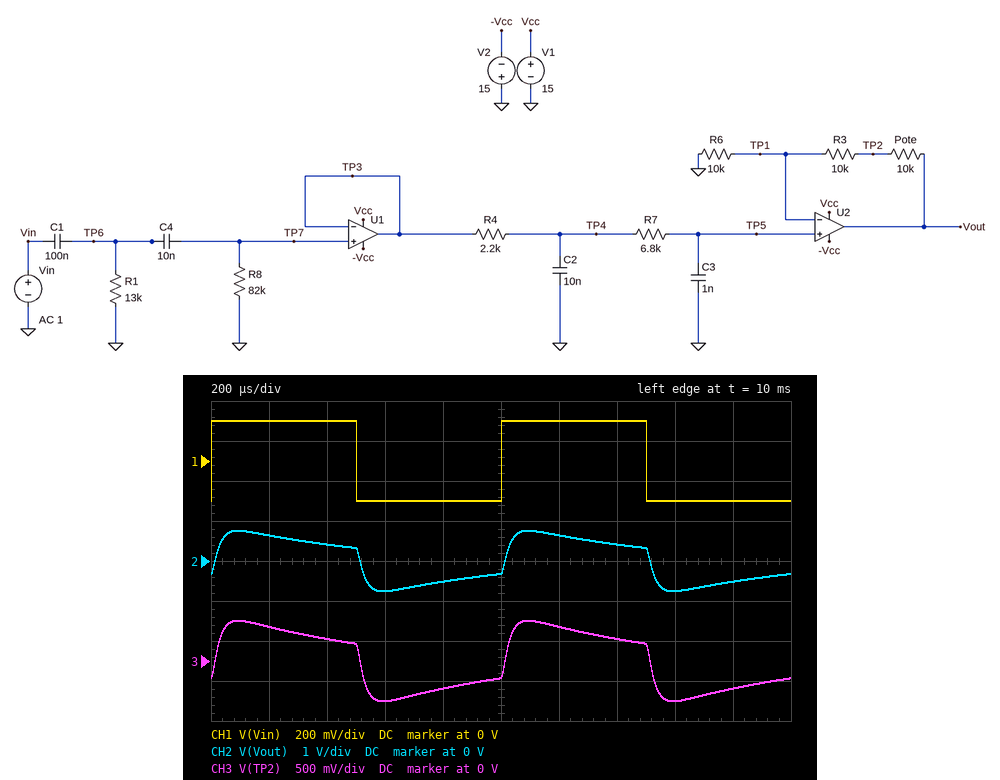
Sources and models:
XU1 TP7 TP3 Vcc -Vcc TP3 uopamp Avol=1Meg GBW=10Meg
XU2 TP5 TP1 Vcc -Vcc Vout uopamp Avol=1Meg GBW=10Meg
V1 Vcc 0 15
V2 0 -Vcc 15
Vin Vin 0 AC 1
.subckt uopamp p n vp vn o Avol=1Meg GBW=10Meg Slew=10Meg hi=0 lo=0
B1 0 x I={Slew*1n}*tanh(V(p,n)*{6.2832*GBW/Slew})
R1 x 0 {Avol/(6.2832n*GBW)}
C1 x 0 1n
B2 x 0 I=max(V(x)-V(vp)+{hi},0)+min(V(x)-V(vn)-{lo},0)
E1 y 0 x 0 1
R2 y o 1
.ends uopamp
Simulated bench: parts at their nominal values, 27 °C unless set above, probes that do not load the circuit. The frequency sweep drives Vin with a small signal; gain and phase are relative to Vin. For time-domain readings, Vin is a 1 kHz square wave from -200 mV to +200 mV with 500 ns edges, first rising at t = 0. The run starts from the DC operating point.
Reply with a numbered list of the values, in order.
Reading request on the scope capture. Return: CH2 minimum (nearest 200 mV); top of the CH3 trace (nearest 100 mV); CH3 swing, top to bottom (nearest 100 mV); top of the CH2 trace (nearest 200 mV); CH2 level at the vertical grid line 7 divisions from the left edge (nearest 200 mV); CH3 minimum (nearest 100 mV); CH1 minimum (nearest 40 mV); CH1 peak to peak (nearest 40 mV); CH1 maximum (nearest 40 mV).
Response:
1. -800 mV
2. 500 mV
3. 1.0 V
4. 800 mV
5. 400 mV
6. -500 mV
7. -200 mV
8. 400 mV
9. 200 mV
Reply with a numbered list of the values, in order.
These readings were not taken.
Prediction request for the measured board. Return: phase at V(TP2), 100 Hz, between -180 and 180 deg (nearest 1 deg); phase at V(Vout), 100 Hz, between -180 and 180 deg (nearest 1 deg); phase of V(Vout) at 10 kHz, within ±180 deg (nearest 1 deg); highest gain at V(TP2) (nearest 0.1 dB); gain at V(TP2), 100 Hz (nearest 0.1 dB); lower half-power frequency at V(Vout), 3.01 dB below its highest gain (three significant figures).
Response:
1. 111 deg
2. 111 deg
3. -76 deg
4. 5.7 dB
5. -5.2 dB
6. 252 Hz
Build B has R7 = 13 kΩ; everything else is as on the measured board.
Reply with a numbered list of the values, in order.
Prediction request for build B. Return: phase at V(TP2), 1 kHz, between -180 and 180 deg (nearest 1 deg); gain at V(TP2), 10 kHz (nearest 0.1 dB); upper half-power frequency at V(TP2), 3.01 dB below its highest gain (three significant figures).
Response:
1. 6 deg
2. -1.4 dB
3. 5.72 kHz
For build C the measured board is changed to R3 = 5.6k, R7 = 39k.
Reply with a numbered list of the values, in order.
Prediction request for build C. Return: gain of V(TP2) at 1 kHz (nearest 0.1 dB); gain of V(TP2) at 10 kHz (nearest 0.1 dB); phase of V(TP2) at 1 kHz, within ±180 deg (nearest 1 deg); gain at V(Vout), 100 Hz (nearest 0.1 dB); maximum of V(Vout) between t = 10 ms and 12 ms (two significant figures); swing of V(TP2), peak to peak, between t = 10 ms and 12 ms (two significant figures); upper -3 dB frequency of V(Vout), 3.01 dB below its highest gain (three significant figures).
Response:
1. 3.2 dB
2. -9.5 dB
3. -3 deg
4. -3.0 dB
5. 580 mV
6. 710 mV
7. 3.54 kHz
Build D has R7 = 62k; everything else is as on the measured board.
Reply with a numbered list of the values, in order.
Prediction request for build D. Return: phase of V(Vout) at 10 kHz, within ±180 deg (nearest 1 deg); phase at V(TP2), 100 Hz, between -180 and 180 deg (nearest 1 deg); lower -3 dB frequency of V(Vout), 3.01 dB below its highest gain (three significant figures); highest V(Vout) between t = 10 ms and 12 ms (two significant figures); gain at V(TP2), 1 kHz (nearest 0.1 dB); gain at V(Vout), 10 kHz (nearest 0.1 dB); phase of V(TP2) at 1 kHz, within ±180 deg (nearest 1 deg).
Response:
1. -127 deg
2. 109 deg
3. 229 Hz
4. 630 mV
5. 5.0 dB
6. -7.3 dB
7. -11 deg
